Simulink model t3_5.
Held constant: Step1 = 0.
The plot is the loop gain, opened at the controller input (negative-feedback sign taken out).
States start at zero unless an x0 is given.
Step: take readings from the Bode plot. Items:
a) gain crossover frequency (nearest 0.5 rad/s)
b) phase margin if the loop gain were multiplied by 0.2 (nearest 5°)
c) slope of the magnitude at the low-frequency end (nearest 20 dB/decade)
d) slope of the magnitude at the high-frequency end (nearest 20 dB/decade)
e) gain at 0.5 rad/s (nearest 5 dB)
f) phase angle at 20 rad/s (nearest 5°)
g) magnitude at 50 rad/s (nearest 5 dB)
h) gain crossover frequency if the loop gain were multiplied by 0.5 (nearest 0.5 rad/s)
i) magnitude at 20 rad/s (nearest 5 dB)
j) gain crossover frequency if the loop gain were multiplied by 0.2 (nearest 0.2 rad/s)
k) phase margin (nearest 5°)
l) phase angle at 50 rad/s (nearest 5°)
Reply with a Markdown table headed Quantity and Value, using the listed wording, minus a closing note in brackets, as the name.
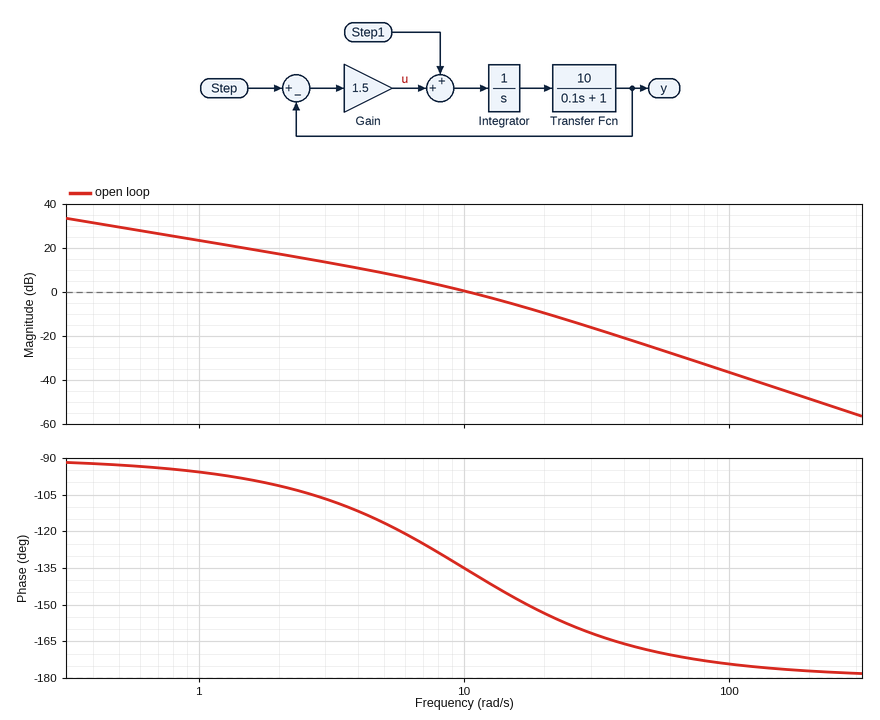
| Quantity | Value |
|---|---|
| gain crossover frequency | 10.5 rad/s |
| phase margin if the loop gain were multiplied by 0.2 | 75° |
| slope of the magnitude at the low-frequency end | -20 dB/decade |
| slope of the magnitude at the high-frequency end | -40 dB/decade |
| gain at 0.5 rad/s | 30 dB |
| phase angle at 20 rad/s | -155° |
| magnitude at 50 rad/s | -25 dB |
| gain crossover frequency if the loop gain were multiplied by 0.5 | 6.5 rad/s |
| magnitude at 20 rad/s | -10 dB |
| gain crossover frequency if the loop gain were multiplied by 0.2 | 2.8 rad/s |
| phase margin | 45° |
| phase angle at 50 rad/s | -170° |
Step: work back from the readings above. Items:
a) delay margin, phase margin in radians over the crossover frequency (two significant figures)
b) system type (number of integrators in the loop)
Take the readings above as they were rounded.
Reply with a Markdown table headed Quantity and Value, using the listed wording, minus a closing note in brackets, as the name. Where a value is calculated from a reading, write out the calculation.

| Quantity | Value |
|---|---|
| delay margin, phase margin in radians over the crossover frequency | 45 × π / 180 / 10.5 = 0.075 s |
| system type | 1 |
